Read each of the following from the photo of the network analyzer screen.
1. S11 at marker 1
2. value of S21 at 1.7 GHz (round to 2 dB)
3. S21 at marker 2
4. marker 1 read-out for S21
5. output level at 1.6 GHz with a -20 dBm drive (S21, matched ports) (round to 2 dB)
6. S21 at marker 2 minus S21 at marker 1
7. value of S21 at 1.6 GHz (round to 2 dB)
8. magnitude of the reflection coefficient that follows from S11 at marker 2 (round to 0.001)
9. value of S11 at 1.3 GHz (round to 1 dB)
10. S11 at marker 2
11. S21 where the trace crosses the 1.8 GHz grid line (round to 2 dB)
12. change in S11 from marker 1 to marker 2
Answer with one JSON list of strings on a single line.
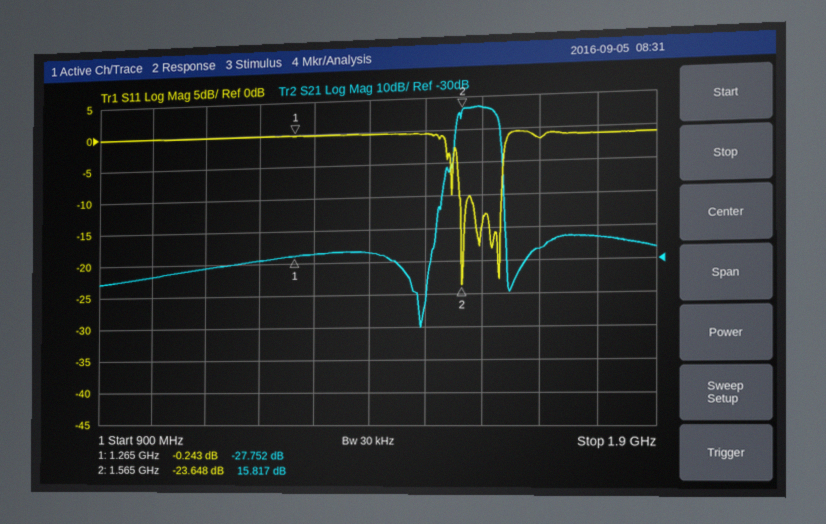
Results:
["-0.243 dB", "-26 dB", "15.817 dB", "-27.752 dB", "-4 dBm", "43.569 dB", "16 dB", "0.066", "0 dB", "-23.648 dB", "-24 dB", "-23.405 dB"]
